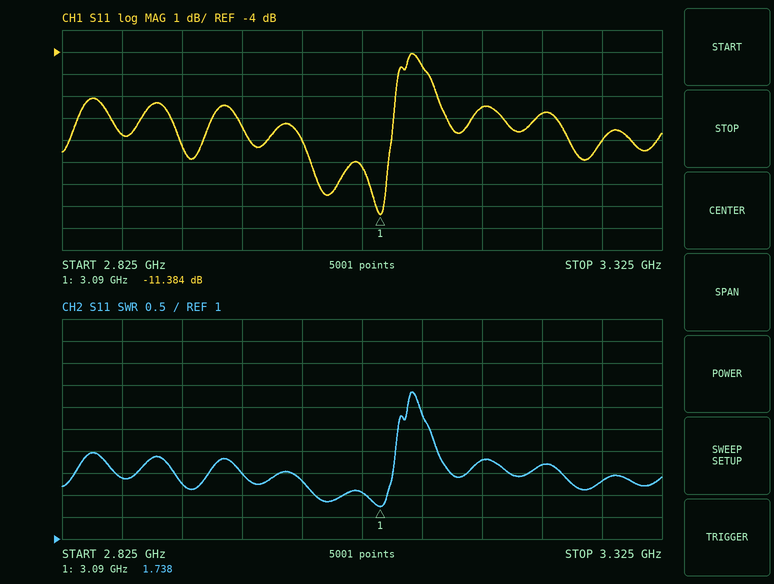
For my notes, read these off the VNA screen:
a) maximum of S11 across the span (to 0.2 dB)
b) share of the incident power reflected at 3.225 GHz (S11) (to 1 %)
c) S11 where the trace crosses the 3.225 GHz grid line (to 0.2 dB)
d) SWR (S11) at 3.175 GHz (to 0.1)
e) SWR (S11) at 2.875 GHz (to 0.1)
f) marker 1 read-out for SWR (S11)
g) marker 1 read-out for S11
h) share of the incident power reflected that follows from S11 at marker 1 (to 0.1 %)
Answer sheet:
-4.0 dB
21 %
-6.8 dB
2.8
2.4
1.738
-11.384 dB
7.3 %
